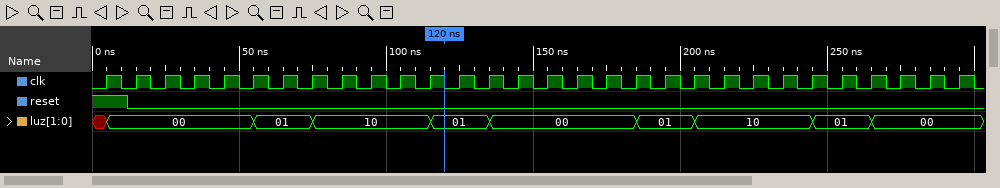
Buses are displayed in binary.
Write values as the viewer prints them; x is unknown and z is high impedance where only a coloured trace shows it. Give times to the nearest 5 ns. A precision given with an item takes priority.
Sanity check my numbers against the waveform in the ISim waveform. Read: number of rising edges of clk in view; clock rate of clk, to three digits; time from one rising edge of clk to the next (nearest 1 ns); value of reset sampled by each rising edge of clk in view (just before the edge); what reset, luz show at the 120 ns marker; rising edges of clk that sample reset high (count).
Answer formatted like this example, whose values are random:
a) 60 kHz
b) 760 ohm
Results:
a) 30
b) 100 MHz
c) 10 ns
d) 1 0 0 0 0 0 0 0 0 0 0 0 0 0 0 0 0 0 0 0 0 0 0 0 0 0 0 0 0 0
e) reset=0, luz=01
f) 1
